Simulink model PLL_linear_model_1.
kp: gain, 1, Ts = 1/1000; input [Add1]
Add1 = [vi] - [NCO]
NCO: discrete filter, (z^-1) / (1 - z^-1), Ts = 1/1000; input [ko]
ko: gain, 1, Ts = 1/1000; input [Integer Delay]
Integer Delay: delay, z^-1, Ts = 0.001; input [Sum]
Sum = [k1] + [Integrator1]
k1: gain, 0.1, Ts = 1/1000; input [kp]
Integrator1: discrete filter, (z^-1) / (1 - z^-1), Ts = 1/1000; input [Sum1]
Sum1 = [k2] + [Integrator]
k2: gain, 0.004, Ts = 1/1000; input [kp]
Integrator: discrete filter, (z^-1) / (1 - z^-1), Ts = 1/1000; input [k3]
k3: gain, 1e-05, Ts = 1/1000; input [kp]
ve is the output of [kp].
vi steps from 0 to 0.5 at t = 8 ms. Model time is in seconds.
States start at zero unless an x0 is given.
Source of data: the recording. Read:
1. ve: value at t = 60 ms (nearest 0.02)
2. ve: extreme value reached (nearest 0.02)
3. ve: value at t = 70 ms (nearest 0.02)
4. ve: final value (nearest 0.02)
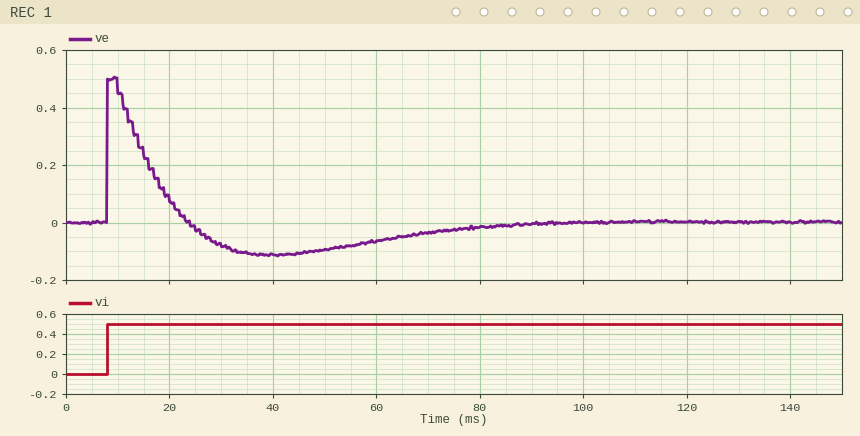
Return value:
-0.06
0.50
-0.04
0.00
